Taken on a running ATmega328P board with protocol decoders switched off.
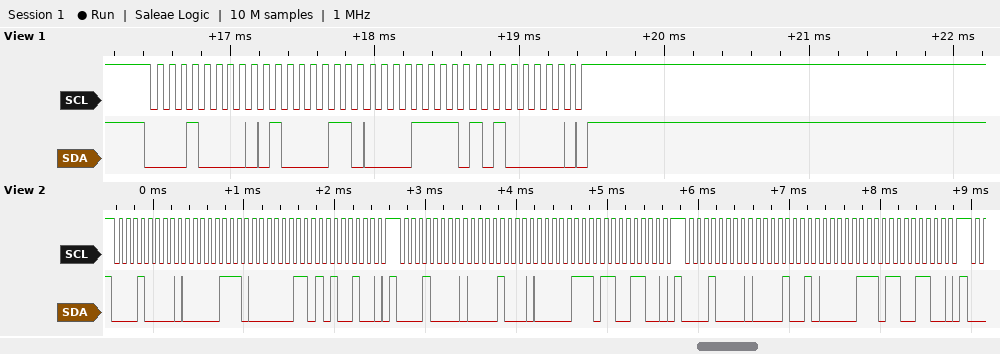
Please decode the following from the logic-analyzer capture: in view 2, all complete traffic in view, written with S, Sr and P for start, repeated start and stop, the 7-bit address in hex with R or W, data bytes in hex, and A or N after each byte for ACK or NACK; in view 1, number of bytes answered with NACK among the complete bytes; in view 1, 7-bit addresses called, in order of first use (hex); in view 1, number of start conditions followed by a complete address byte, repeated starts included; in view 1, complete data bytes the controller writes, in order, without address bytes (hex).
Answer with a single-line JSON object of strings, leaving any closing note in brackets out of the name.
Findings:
{"in view 2, all complete traffic in view, written with S, Sr and P for start, repeated start and stop, the 7-bit address in hex with R or W, data bytes in hex, and A or N after each byte for ACK or NACK": "S 08W A 07 A 03 A A4 A P S 08W A 08 A 07 A CC A P S 08W A 09 A 07 A CC A P", "in view 1, number of bytes answered with NACK among the complete bytes": "0", "in view 1, 7-bit addresses called, in order of first use": "0x08", "in view 1, number of start conditions followed by a complete address byte, repeated starts included": "1", "in view 1, complete data bytes the controller writes, in order, without address bytes": "43 0F A0"}
